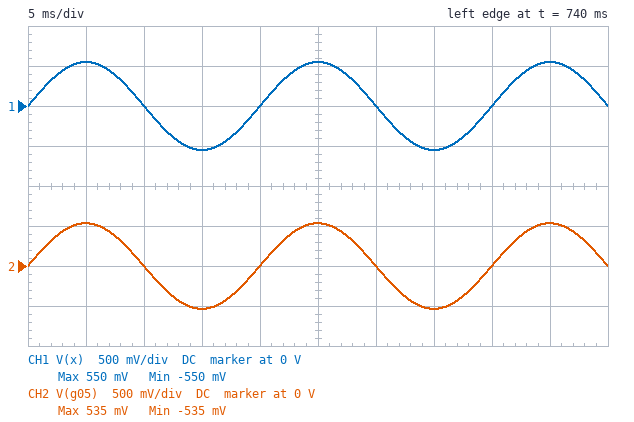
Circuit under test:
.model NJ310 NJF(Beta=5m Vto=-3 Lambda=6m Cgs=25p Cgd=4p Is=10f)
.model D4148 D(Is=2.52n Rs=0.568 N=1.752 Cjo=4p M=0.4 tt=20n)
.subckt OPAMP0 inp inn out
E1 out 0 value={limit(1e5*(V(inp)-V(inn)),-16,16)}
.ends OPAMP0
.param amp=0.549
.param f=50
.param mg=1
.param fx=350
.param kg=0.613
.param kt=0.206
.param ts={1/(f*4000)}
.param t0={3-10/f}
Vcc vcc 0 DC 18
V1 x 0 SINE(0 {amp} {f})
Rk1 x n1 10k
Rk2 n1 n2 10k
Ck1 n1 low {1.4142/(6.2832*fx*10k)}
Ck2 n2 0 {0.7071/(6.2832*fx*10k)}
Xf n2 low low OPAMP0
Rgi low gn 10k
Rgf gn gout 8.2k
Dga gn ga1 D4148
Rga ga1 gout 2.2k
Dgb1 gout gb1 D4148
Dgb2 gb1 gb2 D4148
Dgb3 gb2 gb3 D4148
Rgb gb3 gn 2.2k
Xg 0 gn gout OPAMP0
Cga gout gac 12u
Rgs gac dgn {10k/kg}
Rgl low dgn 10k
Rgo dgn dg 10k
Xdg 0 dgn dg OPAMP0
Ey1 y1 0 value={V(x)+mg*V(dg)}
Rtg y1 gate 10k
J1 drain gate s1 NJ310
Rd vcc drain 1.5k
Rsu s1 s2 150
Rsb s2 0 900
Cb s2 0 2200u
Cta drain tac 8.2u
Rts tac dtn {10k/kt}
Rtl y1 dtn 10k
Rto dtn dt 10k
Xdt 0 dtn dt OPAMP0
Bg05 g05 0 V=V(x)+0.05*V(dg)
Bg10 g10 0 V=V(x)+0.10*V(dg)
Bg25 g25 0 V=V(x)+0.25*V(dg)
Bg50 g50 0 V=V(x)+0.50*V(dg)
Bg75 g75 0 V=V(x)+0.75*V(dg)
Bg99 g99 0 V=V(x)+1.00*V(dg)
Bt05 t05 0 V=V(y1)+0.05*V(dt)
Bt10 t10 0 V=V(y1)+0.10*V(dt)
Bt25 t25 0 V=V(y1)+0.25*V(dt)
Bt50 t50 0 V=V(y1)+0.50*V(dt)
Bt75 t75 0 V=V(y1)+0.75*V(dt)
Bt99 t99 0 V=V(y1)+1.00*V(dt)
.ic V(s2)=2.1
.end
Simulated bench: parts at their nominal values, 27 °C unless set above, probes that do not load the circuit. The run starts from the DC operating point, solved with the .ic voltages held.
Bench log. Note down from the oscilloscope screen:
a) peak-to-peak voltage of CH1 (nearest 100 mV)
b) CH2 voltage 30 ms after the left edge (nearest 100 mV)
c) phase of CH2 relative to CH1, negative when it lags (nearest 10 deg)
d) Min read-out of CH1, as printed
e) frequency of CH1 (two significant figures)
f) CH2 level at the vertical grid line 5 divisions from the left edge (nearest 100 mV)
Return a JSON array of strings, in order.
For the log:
["1.1 V", "0 V", "0 deg", "-550 mV", "50 Hz", "500 mV"]
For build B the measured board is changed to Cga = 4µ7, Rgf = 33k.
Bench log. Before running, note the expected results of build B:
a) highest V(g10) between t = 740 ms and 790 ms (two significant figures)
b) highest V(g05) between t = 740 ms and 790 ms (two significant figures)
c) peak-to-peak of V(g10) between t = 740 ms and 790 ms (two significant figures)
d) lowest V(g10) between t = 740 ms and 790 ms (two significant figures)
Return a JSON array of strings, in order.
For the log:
["540 mV", "550 mV", "1.1 V", "-560 mV"]
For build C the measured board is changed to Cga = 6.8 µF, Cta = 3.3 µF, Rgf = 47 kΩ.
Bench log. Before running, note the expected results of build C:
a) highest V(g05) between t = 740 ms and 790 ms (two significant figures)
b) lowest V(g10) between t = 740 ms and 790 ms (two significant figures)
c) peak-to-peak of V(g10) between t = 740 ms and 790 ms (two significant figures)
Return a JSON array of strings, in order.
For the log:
["550 mV", "-560 mV", "1.1 V"]
